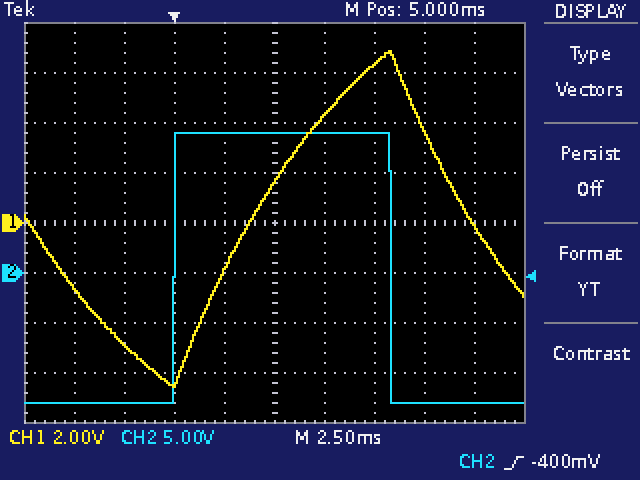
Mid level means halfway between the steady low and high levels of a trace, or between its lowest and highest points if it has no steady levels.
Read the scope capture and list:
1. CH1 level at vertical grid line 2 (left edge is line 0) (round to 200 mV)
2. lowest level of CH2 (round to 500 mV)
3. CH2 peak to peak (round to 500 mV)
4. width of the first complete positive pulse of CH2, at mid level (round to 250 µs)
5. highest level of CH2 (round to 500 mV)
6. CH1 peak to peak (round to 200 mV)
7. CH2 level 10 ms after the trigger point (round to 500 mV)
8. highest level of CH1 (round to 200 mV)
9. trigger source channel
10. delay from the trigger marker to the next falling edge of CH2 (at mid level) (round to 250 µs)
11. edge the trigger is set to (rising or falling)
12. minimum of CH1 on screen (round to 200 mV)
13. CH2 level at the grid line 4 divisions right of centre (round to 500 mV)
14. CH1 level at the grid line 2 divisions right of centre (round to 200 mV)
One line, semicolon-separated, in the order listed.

-4.8 V; -13.0 V; 27.0 V; 10.75 ms; 14.0 V; 13.4 V; 14.0 V; 6.8 V; CH2; 10.75 ms; rising; -6.6 V; -13.0 V; 6.4 V
